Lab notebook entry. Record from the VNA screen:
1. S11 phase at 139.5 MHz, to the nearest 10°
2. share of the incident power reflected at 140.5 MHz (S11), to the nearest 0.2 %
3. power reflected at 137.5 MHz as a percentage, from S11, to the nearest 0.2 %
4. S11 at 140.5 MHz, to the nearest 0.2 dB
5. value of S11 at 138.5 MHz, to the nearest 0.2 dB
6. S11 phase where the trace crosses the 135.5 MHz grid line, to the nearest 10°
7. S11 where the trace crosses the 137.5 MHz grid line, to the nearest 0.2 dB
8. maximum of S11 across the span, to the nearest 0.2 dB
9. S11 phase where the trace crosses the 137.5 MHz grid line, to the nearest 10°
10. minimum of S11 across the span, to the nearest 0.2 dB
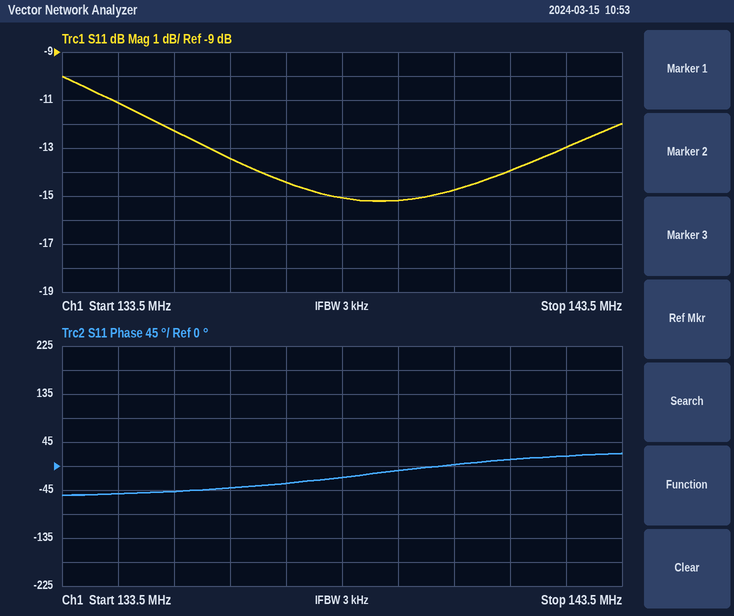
-10°
3.4 %
3.6 %
-14.8 dB
-15.0 dB
-50°
-14.4 dB
-10.0 dB
-30°
-15.2 dB
